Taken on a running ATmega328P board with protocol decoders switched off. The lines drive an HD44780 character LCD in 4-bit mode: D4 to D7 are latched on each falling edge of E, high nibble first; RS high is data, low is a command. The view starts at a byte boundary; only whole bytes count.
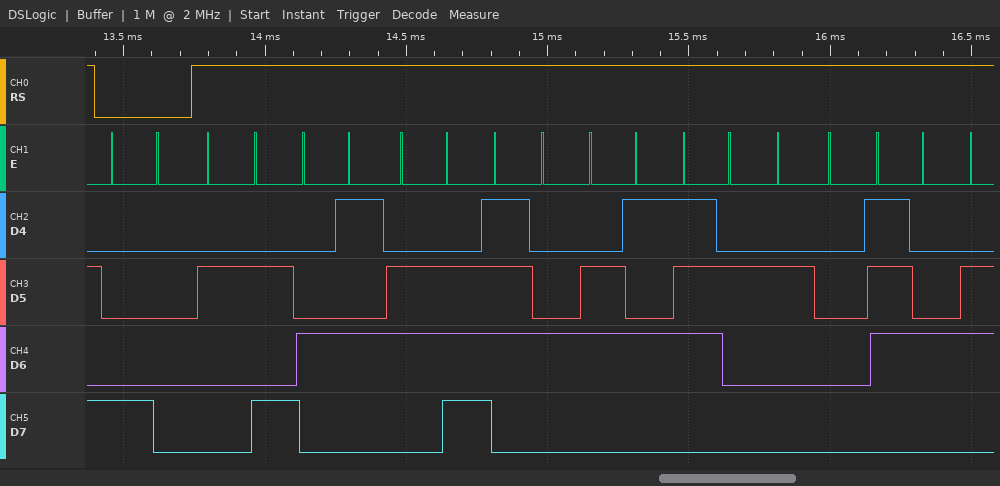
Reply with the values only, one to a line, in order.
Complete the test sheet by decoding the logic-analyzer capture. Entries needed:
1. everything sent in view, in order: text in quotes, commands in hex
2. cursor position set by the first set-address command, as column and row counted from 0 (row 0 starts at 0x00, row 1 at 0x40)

0x80 "*Enter t"
column 0, row 0
